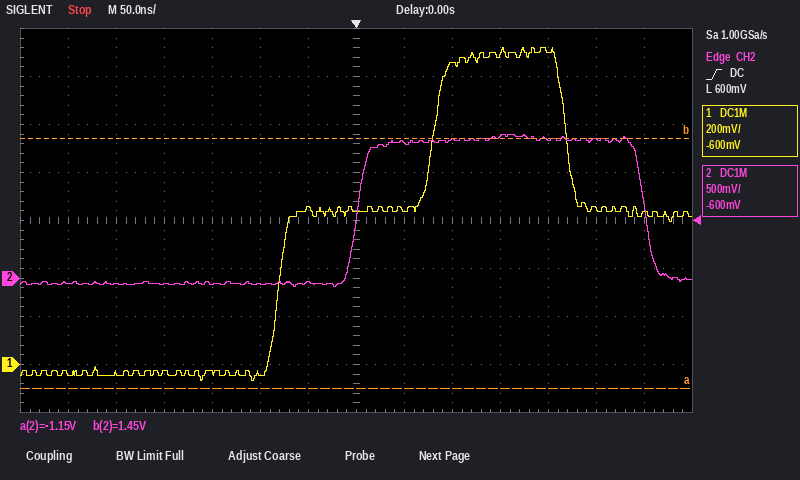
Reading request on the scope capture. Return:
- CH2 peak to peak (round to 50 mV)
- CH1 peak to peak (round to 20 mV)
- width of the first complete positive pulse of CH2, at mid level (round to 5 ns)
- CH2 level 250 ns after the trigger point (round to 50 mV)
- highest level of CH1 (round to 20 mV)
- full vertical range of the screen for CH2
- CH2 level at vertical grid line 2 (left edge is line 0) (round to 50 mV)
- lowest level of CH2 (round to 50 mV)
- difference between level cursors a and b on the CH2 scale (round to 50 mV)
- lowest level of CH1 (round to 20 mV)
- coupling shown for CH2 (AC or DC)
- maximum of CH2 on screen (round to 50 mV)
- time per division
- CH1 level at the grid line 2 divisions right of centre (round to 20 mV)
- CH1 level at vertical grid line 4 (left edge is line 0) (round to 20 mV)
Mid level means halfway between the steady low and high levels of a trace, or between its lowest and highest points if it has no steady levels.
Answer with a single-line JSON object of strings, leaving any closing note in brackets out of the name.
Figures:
{"CH2 peak to peak": "1.60 V", "CH1 peak to peak": "1.38 V", "width of the first complete positive pulse of CH2, at mid level": "300 ns", "CH2 level 250 ns after the trigger point": "1.45 V", "highest level of CH1": "1.32 V", "full vertical range of the screen for CH2": "4 V", "CH2 level at vertical grid line 2 (left edge is line 0)": "-50 mV", "lowest level of CH2": "-100 mV", "difference between level cursors a and b on the CH2 scale": "2.60 V", "lowest level of CH1": "-60 mV", "coupling shown for CH2": "DC", "maximum of CH2 on screen": "1.50 V", "time per division": "50 ns", "CH1 level at the grid line 2 divisions right of centre": "1.26 V", "CH1 level at vertical grid line 4 (left edge is line 0)": "-40 mV"}
